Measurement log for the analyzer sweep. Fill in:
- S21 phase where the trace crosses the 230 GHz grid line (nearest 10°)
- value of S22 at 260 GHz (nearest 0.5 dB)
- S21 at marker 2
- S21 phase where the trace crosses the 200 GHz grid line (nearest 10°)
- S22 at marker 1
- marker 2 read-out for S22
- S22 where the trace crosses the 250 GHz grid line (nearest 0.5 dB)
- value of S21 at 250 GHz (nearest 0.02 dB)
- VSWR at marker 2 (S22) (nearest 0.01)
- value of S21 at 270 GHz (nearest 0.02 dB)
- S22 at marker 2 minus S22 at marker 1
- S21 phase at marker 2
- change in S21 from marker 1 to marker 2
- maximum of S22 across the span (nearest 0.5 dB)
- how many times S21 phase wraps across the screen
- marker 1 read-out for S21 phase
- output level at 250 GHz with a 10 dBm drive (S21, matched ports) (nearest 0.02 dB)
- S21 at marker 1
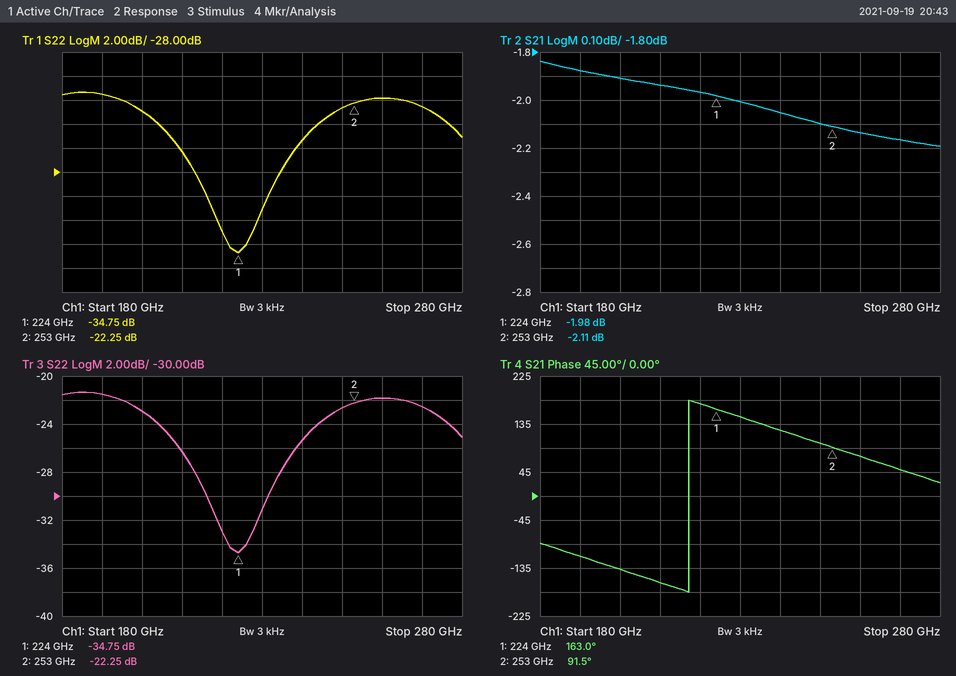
150°
-22.0 dB
-2.11 dB
-140°
-34.75 dB
-22.25 dB
-22.5 dB
-2.10 dB
1.17
-2.16 dB
12.50 dB
91.5°
-0.13 dB
-21.5 dB
1
163.0°
7.90 dBm
-1.98 dB
